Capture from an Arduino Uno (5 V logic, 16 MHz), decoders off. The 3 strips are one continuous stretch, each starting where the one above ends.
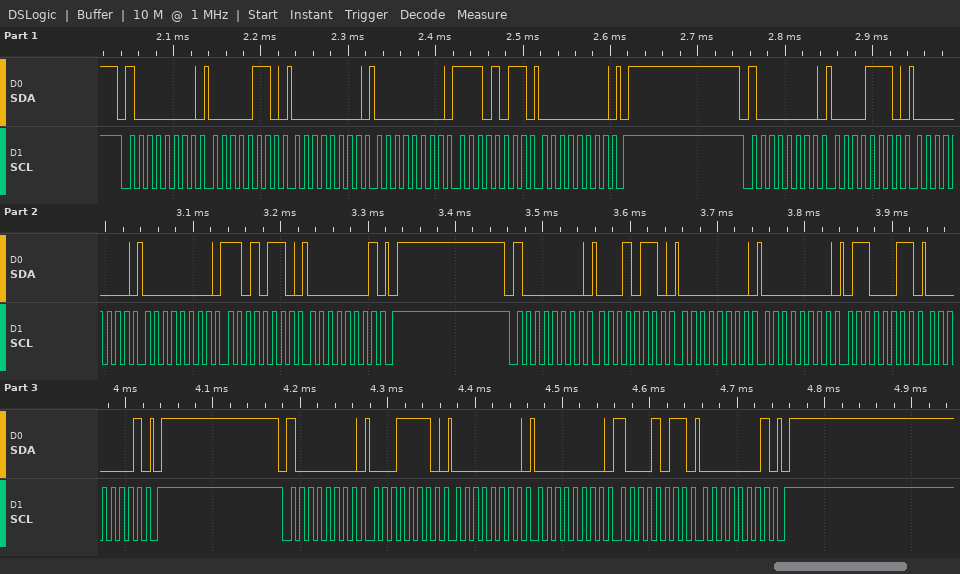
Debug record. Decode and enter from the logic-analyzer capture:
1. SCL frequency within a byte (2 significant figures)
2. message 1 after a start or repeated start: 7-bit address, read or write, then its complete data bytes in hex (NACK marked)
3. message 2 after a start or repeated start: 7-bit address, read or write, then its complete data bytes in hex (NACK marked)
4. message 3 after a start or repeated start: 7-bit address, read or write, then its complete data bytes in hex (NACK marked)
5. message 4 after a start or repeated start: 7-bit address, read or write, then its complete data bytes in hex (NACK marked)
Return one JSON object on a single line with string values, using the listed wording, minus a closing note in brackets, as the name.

{"SCL frequency within a byte": "100 kHz", "message 1 after a start or repeated start: 7-bit address, read or write, then its complete data bytes in hex": "0x40 write: 06 00 00 EB 00", "message 2 after a start or repeated start: 7-bit address, read or write, then its complete data bytes in hex": "0x40 write: 0E 00 00 D6 01", "message 3 after a start or repeated start: 7-bit address, read or write, then its complete data bytes in hex": "0x40 write: 16 00 00 63 01", "message 4 after a start or repeated start: 7-bit address, read or write, then its complete data bytes in hex": "0x40 write: 1E 00 00 8B 01"}
